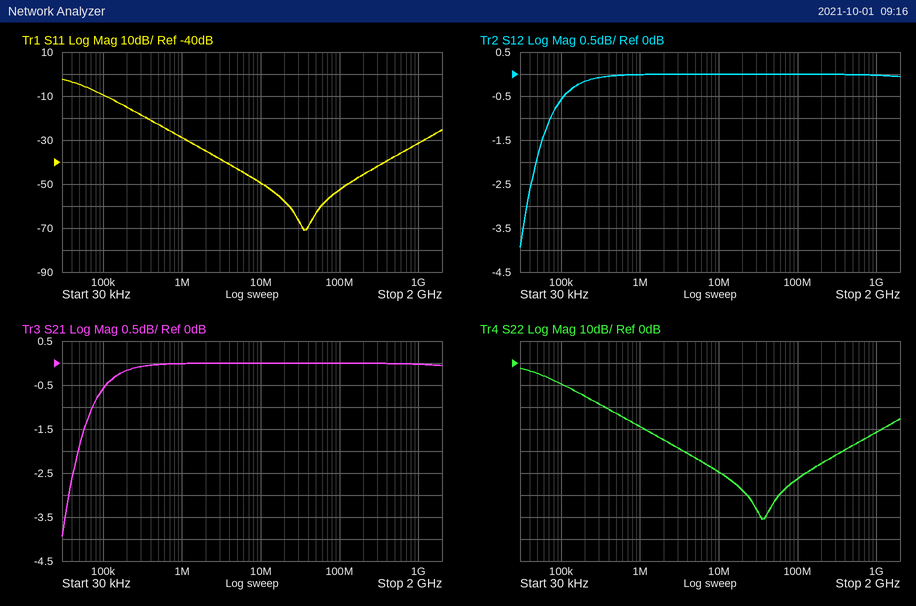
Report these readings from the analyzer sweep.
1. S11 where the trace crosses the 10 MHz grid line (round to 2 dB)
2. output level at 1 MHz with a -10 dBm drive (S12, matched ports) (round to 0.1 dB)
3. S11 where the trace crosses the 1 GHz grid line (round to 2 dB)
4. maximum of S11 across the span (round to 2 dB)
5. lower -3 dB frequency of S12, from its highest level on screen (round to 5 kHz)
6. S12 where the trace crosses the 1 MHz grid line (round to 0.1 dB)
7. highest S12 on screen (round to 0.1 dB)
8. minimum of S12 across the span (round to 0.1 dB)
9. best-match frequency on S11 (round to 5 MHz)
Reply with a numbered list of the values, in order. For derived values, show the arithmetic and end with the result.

1. -50 dB
2. -10 dBm + (0.0 dB) = -10.0 dBm
3. -32 dB
4. -2 dB
5. 35 kHz
6. 0.0 dB
7. 0.0 dB
8. -3.9 dB
9. 35 MHz
